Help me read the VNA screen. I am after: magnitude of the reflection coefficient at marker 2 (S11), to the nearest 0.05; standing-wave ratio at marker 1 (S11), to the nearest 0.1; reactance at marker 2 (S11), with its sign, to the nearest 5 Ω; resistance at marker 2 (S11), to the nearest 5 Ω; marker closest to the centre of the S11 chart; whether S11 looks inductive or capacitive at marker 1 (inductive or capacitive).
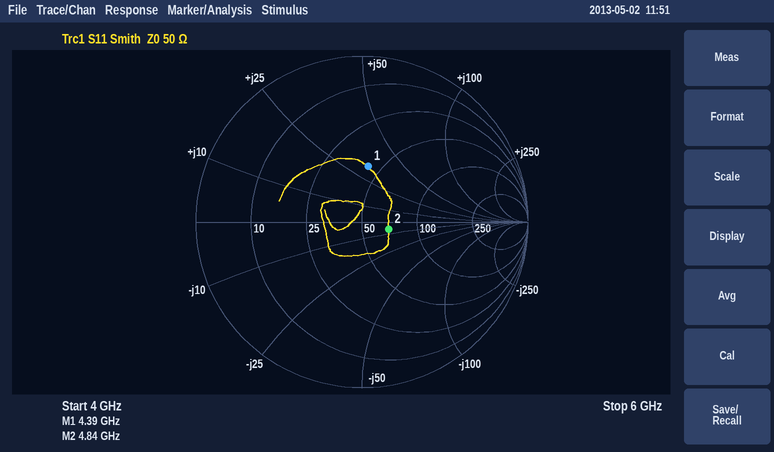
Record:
0.15
2.0
-5 Ω
70 Ω
marker 2
inductive
